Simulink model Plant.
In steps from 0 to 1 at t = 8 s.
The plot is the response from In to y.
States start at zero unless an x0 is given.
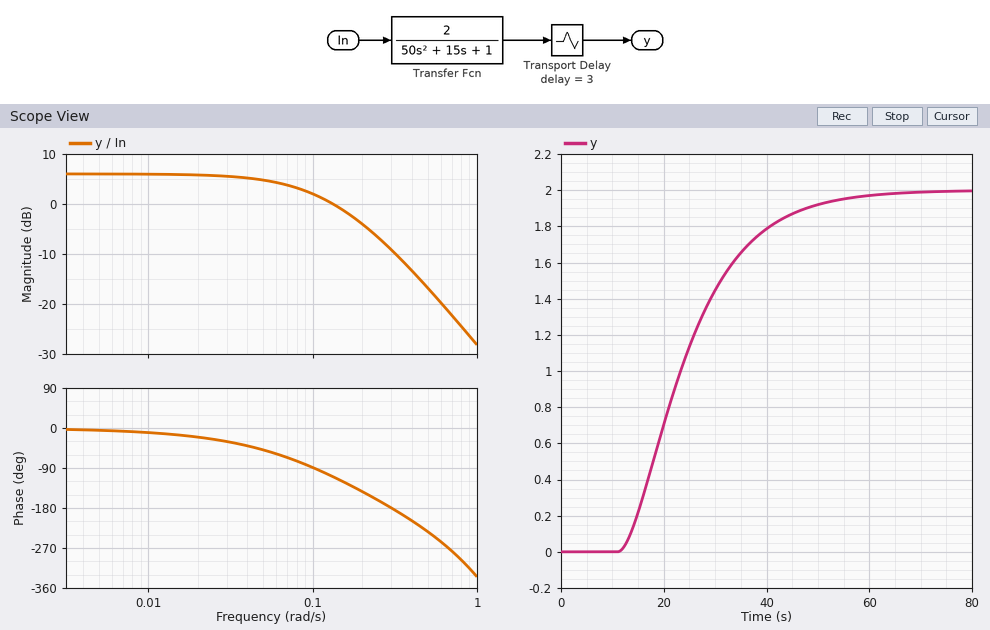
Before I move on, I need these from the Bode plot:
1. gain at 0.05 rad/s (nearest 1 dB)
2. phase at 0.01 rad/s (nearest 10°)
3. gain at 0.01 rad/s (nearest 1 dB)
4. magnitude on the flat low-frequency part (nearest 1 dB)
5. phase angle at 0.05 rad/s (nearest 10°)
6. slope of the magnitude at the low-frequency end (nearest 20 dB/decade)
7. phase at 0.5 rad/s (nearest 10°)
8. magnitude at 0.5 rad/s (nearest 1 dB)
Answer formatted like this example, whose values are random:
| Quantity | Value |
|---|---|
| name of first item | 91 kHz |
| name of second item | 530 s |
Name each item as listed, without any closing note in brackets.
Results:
| Quantity | Value |
|---|---|
| gain at 0.05 rad/s | 5 dB |
| phase at 0.01 rad/s | -10° |
| gain at 0.01 rad/s | 6 dB |
| magnitude on the flat low-frequency part | 6 dB |
| phase angle at 0.05 rad/s | -50° |
| slope of the magnitude at the low-frequency end | 0 dB/decade |
| phase at 0.5 rad/s | -230° |
| magnitude at 0.5 rad/s | -17 dB |
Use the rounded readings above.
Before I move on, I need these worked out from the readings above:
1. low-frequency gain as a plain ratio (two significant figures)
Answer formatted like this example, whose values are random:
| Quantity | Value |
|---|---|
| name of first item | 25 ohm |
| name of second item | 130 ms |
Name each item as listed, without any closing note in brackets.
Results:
| Quantity | Value |
|---|---|
| low-frequency gain as a plain ratio | 2.0 |
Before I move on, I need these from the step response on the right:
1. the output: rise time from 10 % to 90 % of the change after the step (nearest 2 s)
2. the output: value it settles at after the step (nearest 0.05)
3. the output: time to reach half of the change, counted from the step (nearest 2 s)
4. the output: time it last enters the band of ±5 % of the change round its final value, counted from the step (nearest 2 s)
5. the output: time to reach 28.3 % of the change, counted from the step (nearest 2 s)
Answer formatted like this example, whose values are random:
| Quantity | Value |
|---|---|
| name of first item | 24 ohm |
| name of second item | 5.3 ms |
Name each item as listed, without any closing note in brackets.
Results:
| Quantity | Value |
|---|---|
| the output: rise time from 10 % to 90 % of the change after the step | 26 s |
| the output: value it settles at after the step | 2.00 |
| the output: time to reach half of the change, counted from the step | 16 s |
| the output: time it last enters the band of ±5 % of the change round its final value, counted from the step | 40 s |
| the output: time to reach 28.3 % of the change, counted from the step | 10 s |
